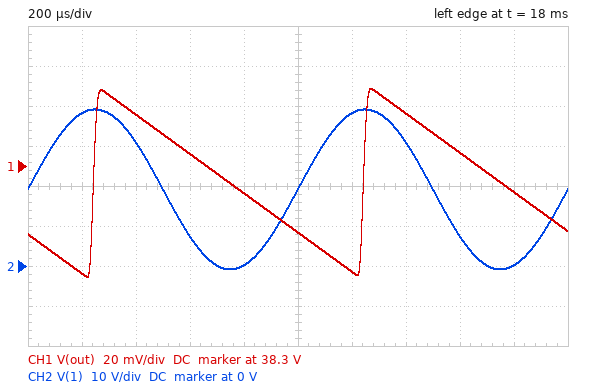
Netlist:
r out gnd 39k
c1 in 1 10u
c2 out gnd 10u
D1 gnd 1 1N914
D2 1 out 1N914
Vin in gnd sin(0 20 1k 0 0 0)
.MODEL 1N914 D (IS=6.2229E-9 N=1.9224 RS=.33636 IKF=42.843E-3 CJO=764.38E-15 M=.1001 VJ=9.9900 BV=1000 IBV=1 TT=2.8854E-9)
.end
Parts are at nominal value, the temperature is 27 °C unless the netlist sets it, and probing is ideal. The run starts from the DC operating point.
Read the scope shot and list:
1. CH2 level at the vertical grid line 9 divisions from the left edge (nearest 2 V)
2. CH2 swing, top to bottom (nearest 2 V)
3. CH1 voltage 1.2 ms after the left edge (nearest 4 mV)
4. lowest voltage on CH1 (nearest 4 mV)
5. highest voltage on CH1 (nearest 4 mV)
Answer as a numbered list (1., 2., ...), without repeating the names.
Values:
1. 0 V
2. 40 V
3. 38.248 V
4. 38.244 V
5. 38.340 V
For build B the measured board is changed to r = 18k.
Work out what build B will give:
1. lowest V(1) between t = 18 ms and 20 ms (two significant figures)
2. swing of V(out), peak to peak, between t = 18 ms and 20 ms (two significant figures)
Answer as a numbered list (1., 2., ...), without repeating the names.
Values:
1. -900 mV
2. 200 mV
